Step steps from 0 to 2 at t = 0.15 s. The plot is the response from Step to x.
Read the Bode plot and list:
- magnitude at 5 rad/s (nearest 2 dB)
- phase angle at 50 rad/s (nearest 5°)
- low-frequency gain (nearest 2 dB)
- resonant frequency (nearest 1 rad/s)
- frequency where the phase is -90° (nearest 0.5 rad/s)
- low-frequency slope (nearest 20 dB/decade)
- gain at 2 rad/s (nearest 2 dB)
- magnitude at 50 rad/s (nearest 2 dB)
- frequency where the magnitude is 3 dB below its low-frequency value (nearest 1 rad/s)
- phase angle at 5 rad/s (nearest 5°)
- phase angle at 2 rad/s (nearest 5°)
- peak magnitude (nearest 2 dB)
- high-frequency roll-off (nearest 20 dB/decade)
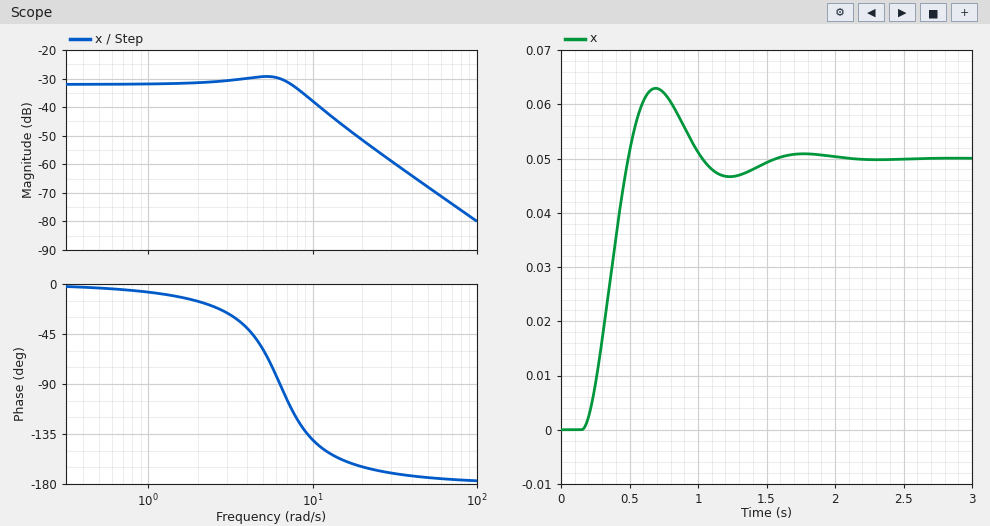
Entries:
-30 dB
-175°
-32 dB
5 rad/s
6.5 rad/s
0 dB/decade
-32 dB
-68 dB
9 rad/s
-60°
-15°
-30 dB
-40 dB/decade
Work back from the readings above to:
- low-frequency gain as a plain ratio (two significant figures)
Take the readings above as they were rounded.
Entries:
0.025
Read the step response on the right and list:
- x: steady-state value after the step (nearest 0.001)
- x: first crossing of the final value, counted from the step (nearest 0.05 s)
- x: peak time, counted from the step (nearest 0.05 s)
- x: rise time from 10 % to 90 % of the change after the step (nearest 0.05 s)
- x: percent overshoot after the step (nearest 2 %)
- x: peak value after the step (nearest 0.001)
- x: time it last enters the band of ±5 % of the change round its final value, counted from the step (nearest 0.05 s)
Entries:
0.050
0.35 s
0.55 s
0.25 s
26 %
0.063
1.20 s
